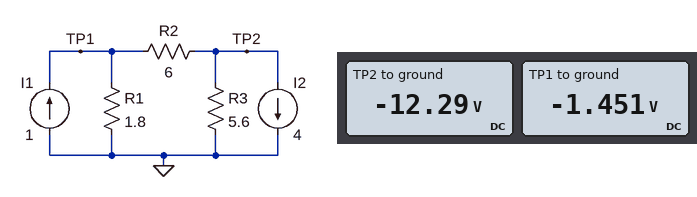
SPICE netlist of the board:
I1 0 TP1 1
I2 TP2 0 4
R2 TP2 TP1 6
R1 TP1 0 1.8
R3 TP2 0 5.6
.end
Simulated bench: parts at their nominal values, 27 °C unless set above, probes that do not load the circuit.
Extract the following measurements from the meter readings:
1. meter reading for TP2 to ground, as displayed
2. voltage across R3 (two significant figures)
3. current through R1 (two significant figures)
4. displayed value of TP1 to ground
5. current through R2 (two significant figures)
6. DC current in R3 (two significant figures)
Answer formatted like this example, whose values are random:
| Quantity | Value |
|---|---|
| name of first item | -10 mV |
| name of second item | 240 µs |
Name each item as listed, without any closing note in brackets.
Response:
| Quantity | Value |
|---|---|
| meter reading for TP2 to ground, as displayed | -12.29 V |
| voltage across R3 | 12 V |
| current through R1 | 810 mA |
| displayed value of TP1 to ground | -1.451 V |
| current through R2 | 1.8 A |
| DC current in R3 | 2.2 A |
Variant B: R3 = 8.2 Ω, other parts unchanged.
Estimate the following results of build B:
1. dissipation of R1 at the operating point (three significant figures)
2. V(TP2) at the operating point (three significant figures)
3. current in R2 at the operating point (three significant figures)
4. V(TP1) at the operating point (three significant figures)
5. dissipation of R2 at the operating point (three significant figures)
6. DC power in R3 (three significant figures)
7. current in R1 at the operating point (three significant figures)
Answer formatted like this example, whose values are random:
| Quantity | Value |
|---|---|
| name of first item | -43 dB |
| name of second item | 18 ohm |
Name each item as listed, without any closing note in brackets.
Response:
| Quantity | Value |
|---|---|
| dissipation of R1 at the operating point | 2.43 W |
| V(TP2) at the operating point | -15.1 V |
| current in R2 at the operating point | 2.16 A |
| V(TP1) at the operating point | -2.09 V |
| dissipation of R2 at the operating point | 28.1 W |
| DC power in R3 | 27.7 W |
| current in R1 at the operating point | 1.16 A |
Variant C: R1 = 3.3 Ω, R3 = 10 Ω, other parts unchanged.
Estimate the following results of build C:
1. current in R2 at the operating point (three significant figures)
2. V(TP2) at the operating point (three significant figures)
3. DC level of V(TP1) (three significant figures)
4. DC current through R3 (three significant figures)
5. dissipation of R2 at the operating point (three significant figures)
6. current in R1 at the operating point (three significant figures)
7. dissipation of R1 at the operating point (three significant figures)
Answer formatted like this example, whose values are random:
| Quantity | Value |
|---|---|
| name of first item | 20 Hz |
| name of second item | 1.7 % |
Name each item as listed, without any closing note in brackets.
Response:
| Quantity | Value |
|---|---|
| current in R2 at the operating point | 2.24 A |
| V(TP2) at the operating point | -17.6 V |
| DC level of V(TP1) | -4.10 V |
| DC current through R3 | 1.76 A |
| dissipation of R2 at the operating point | 30.2 W |
| current in R1 at the operating point | 1.24 A |
| dissipation of R1 at the operating point | 5.10 W |
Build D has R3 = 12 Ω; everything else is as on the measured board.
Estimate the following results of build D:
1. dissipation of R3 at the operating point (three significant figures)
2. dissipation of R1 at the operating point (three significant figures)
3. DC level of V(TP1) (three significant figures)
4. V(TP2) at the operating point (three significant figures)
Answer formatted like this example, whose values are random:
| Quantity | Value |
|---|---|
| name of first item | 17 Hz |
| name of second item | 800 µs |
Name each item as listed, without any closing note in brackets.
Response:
| Quantity | Value |
|---|---|
| dissipation of R3 at the operating point | 26.5 W |
| dissipation of R1 at the operating point | 4.13 W |
| DC level of V(TP1) | -2.73 V |
| V(TP2) at the operating point | -17.8 V |
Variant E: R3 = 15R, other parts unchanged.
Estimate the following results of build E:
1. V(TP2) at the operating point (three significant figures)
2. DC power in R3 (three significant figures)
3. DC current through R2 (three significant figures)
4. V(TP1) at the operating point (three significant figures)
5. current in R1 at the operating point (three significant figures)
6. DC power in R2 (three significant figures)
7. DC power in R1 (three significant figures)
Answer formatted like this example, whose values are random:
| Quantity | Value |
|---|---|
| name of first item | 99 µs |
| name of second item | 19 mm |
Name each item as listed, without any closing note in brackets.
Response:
| Quantity | Value |
|---|---|
| V(TP2) at the operating point | -19.3 V |
| DC power in R3 | 24.9 W |
| DC current through R2 | 2.71 A |
| V(TP1) at the operating point | -3.08 V |
| current in R1 at the operating point | 1.71 A |
| DC power in R2 | 44.1 W |
| DC power in R1 | 5.27 W |
